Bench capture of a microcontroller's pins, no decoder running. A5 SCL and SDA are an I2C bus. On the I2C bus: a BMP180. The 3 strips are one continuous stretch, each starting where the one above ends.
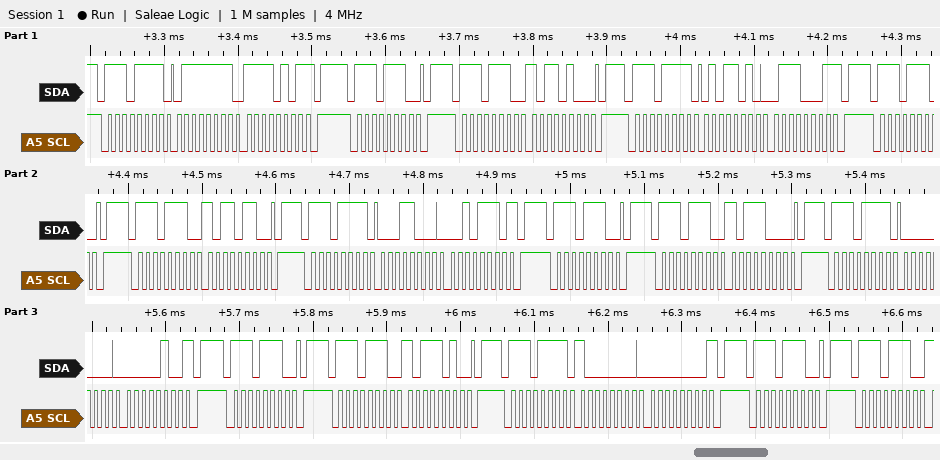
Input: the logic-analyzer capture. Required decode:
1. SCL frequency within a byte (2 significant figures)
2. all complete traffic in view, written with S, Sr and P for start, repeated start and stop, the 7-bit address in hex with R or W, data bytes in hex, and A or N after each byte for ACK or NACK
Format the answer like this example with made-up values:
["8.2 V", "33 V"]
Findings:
["100 kHz", "S 77R A 7F A F5 N P S 77W A P S 77W A B4 A P S 77R A 5A A 71 N P S 77W A P S 77W A B6 A P S 77R A 18 A 2E N P S 77W A P S 77W A B8 A P S 77R A 00 A 04 N P S 77W A P S 77W A BA A P S 77R A 80 A 00 N P S 77W A P S 77W A"]
